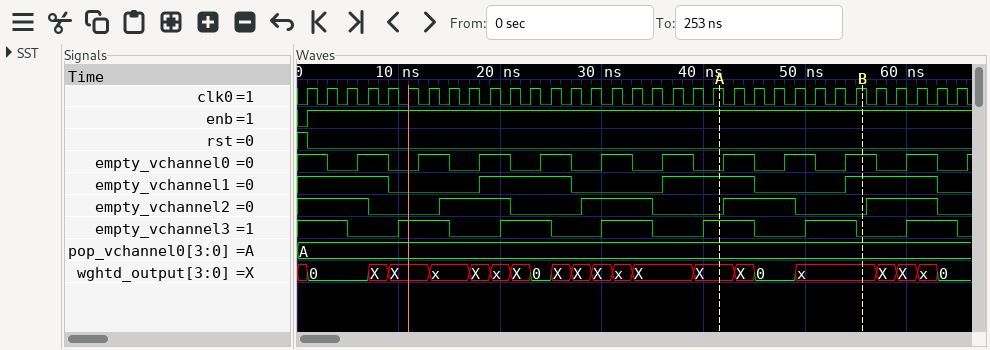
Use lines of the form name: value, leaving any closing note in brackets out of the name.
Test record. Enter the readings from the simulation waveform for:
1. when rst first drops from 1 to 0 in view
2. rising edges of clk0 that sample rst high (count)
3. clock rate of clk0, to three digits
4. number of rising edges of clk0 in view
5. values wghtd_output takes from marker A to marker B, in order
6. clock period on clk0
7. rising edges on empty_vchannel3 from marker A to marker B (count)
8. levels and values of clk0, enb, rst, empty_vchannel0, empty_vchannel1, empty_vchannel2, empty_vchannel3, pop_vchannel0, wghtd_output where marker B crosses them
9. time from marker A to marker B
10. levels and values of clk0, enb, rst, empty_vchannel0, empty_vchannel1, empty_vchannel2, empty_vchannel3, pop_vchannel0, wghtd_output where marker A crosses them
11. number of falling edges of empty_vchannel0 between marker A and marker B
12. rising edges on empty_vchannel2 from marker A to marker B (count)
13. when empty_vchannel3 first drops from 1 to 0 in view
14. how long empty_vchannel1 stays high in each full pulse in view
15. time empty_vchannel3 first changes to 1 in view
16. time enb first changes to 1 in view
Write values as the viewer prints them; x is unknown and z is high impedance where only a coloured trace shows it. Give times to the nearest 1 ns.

when rst first drops from 1 to 0 in view: 1 ns
rising edges of clk0 that sample rst high: 1
clock rate of clk0, to three digits: 500 MHz
number of rising edges of clk0 in view: 33
values wghtd_output takes from marker A to marker B, in order: X, X, 0, x
clock period on clk0: 2 ns
rising edges on empty_vchannel3 from marker A to marker B: 1
levels and values of clk0, enb, rst, empty_vchannel0, empty_vchannel1, empty_vchannel2, empty_vchannel3, pop_vchannel0, wghtd_output where marker B crosses them: clk0=1, enb=1, rst=0, empty_vchannel0=1, empty_vchannel1=1, empty_vchannel2=0, empty_vchannel3=0, pop_vchannel0=A, wghtd_output=x
time from marker A to marker B: 14 ns
levels and values of clk0, enb, rst, empty_vchannel0, empty_vchannel1, empty_vchannel2, empty_vchannel3, pop_vchannel0, wghtd_output where marker A crosses them: clk0=1, enb=1, rst=0, empty_vchannel0=0, empty_vchannel1=1, empty_vchannel2=0, empty_vchannel3=1, pop_vchannel0=A, wghtd_output=X
number of falling edges of empty_vchannel0 between marker A and marker B: 2
rising edges on empty_vchannel2 from marker A to marker B: 1
when empty_vchannel3 first drops from 1 to 0 in view: 5 ns
how long empty_vchannel1 stays high in each full pulse in view: 9 ns, 9 ns, 9 ns
time empty_vchannel3 first changes to 1 in view: 10 ns
time enb first changes to 1 in view: 1 ns
